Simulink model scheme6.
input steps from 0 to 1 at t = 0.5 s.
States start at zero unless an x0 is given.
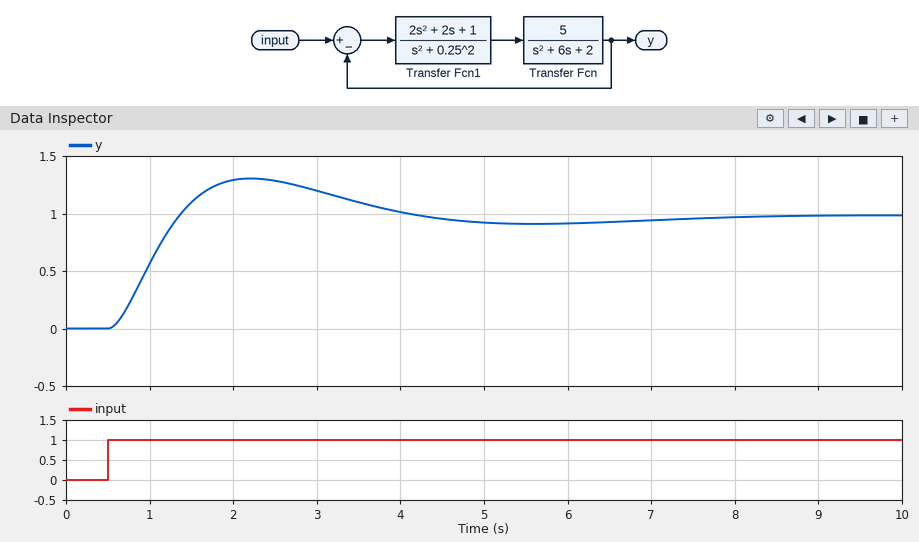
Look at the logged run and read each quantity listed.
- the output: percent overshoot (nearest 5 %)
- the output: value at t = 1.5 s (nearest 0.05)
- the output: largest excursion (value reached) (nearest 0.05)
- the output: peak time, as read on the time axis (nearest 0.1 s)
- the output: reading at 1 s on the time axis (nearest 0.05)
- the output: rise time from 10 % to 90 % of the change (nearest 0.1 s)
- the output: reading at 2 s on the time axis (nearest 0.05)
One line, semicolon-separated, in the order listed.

35 %; 1.10; 1.30; 2.2 s; 0.55; 0.6 s; 1.30
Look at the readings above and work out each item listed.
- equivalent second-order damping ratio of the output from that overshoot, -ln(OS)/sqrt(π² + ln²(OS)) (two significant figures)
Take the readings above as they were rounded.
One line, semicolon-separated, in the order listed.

0.32
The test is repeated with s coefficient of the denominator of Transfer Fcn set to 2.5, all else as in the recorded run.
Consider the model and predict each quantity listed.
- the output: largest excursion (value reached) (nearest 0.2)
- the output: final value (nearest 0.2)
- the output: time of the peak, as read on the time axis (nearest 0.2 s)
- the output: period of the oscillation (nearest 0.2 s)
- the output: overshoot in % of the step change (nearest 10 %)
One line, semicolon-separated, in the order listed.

1.4; 1.0; 1.6 s; 2.0 s; 50 %
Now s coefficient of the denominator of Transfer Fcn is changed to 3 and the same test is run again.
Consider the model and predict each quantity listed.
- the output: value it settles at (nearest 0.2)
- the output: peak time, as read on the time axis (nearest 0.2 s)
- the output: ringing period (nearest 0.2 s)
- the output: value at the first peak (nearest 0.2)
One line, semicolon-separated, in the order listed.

1.0; 1.6 s; 2.0 s; 1.4
